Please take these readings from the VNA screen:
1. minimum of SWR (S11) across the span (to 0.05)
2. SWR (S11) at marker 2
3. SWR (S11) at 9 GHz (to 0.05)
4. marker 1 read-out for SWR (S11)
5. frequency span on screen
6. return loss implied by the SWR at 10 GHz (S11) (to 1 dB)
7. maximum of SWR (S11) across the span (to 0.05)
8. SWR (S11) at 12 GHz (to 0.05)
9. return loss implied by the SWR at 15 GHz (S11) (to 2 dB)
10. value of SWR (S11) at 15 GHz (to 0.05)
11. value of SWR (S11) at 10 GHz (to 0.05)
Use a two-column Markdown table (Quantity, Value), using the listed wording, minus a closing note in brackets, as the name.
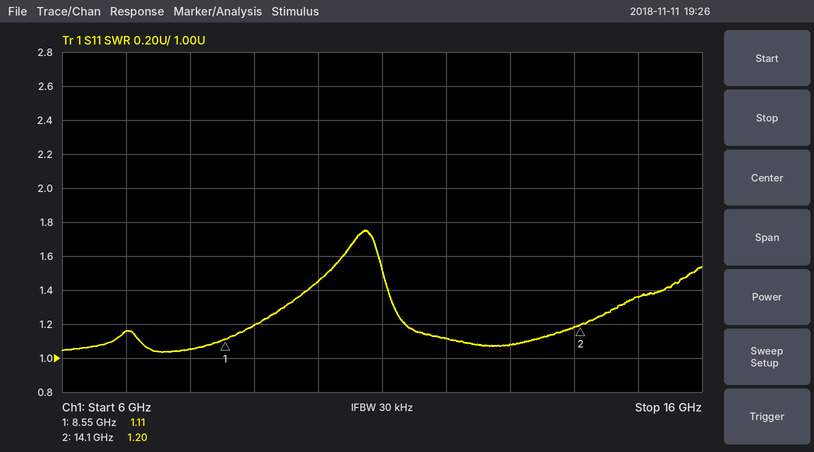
| Quantity | Value |
|---|---|
| minimum of SWR (S11) across the span | 1.05 |
| SWR (S11) at marker 2 | 1.20 |
| SWR (S11) at 9 GHz | 1.20 |
| marker 1 read-out for SWR | 1.11 |
| frequency span on screen | 10 GHz |
| return loss implied by the SWR at 10 GHz (S11) | 15 dB |
| maximum of SWR (S11) across the span | 1.75 |
| SWR (S11) at 12 GHz | 1.10 |
| return loss implied by the SWR at 15 GHz (S11) | 16 dB |
| value of SWR (S11) at 15 GHz | 1.35 |
| value of SWR (S11) at 10 GHz | 1.45 |
